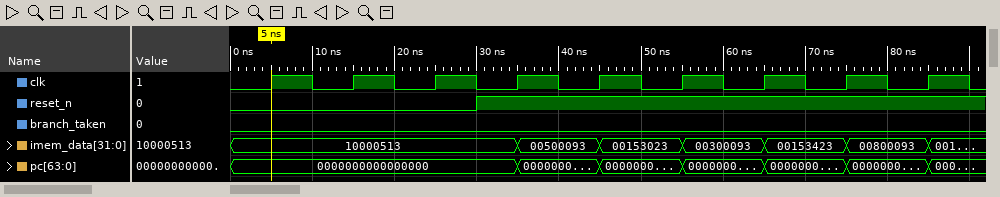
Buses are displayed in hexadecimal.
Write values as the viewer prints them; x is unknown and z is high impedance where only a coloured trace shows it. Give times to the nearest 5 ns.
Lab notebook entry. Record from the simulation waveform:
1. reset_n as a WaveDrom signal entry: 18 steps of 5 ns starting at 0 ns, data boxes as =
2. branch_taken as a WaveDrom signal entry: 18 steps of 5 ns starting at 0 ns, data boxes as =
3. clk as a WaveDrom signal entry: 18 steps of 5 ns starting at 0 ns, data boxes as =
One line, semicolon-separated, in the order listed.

{name: 'reset_n', wave: '0.....1...........'}; {name: 'branch_taken', wave: '0.................'}; {name: 'clk', wave: '010101010101010101'}
